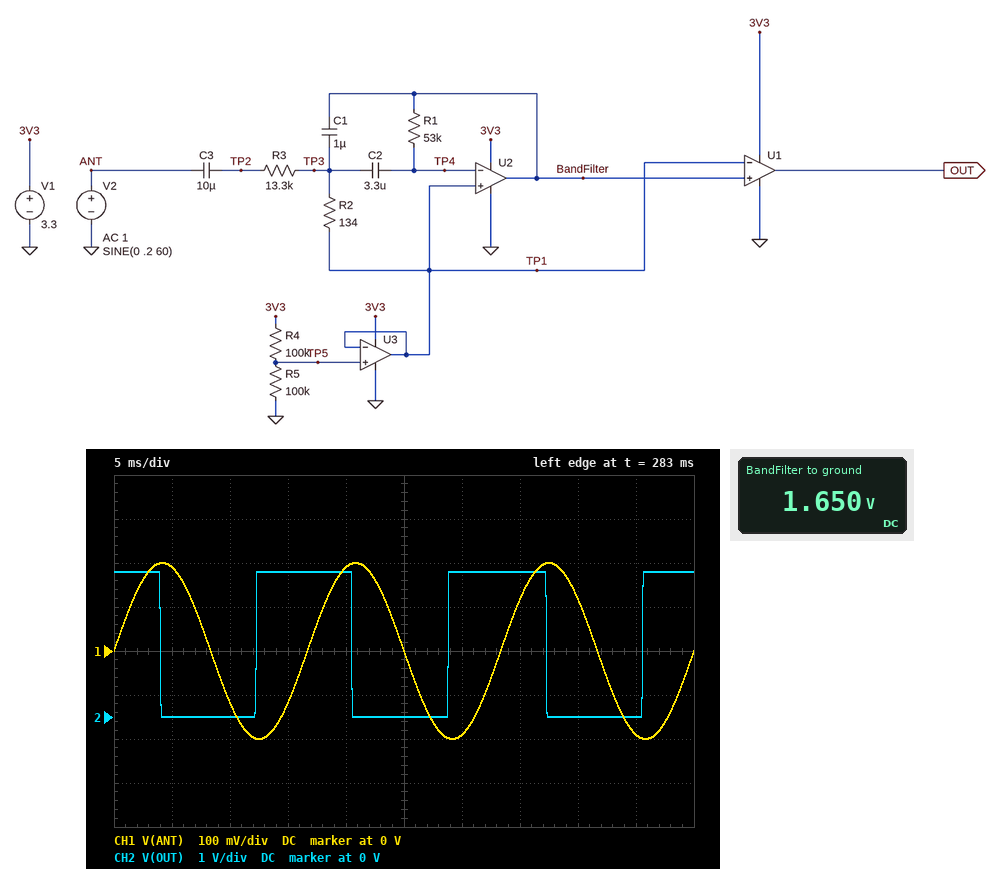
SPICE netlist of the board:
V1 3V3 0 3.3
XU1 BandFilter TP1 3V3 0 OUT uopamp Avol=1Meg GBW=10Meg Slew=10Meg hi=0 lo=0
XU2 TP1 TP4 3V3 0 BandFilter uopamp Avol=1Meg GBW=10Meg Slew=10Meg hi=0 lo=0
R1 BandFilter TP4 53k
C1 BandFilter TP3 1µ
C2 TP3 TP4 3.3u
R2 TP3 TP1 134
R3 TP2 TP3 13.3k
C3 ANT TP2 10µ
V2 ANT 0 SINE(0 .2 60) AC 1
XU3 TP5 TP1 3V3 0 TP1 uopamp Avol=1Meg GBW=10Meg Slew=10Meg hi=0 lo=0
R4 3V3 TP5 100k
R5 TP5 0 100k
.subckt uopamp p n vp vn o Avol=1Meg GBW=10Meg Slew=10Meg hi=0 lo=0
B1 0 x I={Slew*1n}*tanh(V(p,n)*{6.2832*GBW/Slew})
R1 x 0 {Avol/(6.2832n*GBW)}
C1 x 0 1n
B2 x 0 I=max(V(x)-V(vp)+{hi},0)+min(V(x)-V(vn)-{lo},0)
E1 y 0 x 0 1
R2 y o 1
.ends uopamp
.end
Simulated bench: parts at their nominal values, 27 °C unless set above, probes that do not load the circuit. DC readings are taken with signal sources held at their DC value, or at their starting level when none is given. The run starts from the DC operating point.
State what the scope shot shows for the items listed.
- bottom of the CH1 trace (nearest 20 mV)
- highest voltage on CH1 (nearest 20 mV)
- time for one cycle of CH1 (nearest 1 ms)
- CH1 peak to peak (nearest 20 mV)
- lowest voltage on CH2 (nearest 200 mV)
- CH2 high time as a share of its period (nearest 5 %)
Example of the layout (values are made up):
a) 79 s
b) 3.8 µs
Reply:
a) -200 mV
b) 200 mV
c) 17 ms
d) 400 mV
e) 0 V
f) 50 %
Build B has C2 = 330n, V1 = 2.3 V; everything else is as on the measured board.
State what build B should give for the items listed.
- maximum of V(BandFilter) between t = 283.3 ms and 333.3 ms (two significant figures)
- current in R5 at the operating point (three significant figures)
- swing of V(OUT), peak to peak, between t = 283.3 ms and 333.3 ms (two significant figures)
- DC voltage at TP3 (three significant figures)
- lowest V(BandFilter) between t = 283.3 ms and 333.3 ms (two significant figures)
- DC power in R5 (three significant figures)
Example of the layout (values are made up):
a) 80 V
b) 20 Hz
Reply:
a) 1.2 V
b) 11.5 µA
c) 2.3 V
d) 1.15 V
e) 1.1 V
f) 13.2 µW
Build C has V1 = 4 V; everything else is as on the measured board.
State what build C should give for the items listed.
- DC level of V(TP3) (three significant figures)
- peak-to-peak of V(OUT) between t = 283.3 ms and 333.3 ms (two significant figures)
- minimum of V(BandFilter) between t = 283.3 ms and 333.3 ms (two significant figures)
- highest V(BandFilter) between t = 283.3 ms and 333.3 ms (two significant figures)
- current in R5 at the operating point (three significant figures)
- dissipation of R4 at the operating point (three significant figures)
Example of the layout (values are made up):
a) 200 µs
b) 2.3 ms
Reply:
a) 2.00 V
b) 4.0 V
c) 1.9 V
d) 2.1 V
e) 20.0 µA
f) 40.0 µW
